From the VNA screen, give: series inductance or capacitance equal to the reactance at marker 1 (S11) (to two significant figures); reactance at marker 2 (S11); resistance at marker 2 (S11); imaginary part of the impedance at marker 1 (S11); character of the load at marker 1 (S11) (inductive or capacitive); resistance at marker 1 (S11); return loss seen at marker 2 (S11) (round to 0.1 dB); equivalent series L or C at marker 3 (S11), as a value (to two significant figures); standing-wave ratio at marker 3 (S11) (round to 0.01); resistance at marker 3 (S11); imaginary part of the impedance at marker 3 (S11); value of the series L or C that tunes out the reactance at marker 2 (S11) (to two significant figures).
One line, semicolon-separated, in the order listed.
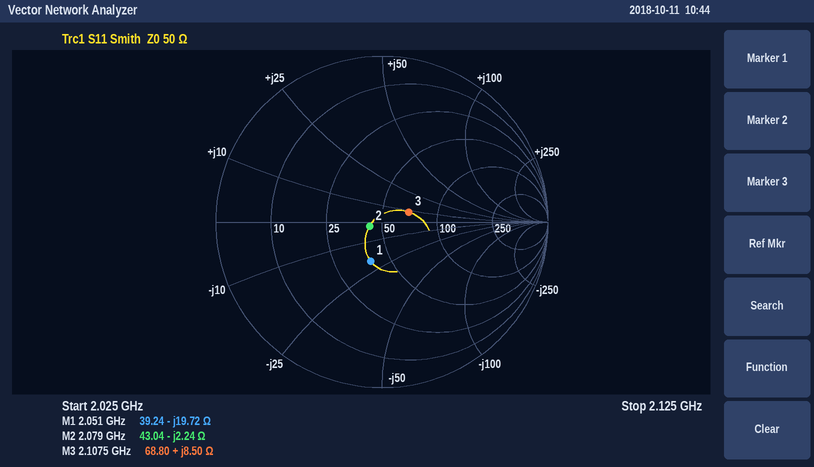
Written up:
3.9 pF; -2.24 Ω; 43.04 Ω; -19.72 Ω; capacitive; 39.24 Ω; 22.1 dB; 640 pH; 1.42; 68.80 Ω; +8.50 Ω; 170 pH
